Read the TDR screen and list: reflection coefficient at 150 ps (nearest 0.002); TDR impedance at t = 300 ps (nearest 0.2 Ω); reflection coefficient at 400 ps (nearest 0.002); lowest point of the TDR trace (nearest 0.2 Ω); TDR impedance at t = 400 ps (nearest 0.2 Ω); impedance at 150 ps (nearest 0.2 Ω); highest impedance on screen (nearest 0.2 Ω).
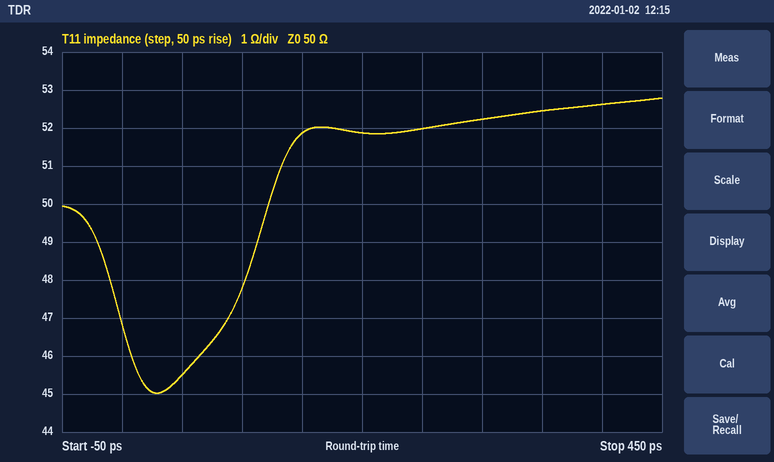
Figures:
+0.018
52.2 Ω
+0.026
45.0 Ω
52.6 Ω
51.8 Ω
52.8 Ω
